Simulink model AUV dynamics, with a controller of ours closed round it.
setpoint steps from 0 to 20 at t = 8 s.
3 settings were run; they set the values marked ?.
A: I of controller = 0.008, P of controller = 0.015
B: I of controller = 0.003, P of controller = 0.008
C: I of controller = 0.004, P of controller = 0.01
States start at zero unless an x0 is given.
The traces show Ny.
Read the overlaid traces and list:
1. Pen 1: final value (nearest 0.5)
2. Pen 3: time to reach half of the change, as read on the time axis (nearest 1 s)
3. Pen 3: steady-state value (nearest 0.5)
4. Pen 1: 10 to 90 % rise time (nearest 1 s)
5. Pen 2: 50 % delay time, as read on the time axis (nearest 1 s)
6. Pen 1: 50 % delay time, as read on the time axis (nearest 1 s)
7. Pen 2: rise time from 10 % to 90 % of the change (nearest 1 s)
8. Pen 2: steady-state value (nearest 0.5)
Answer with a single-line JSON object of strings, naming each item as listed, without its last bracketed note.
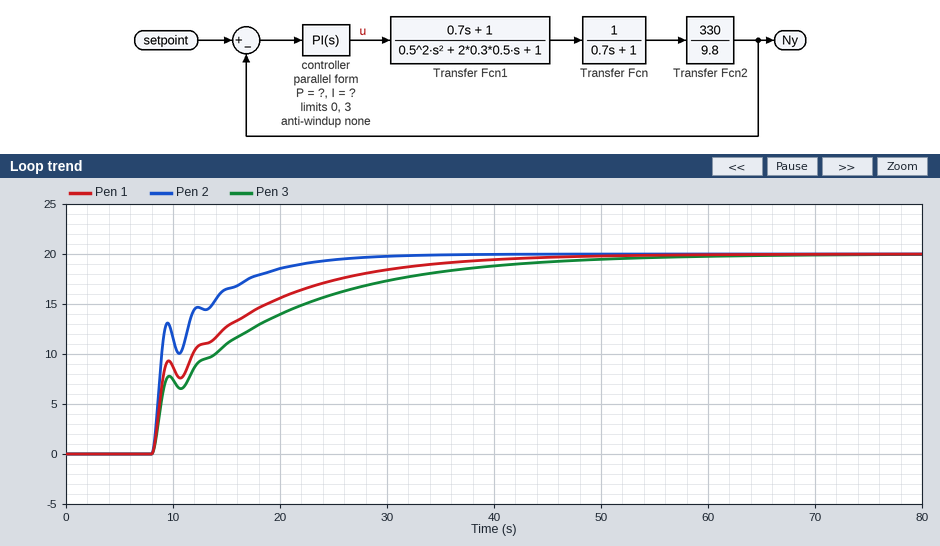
{"Pen 1: final value": "20.0", "Pen 3: time to reach half of the change, as read on the time axis": "14 s", "Pen 3: steady-state value": "20.0", "Pen 1: 10 to 90 % rise time": "19 s", "Pen 2: 50 % delay time, as read on the time axis": "9 s", "Pen 1: 50 % delay time, as read on the time axis": "12 s", "Pen 2: rise time from 10 % to 90 % of the change": "10 s", "Pen 2: steady-state value": "20.0"}
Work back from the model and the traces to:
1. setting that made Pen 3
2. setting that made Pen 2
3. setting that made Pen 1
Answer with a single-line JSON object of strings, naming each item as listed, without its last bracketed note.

{"setting that made Pen 3": "B", "setting that made Pen 2": "A", "setting that made Pen 1": "C"}
